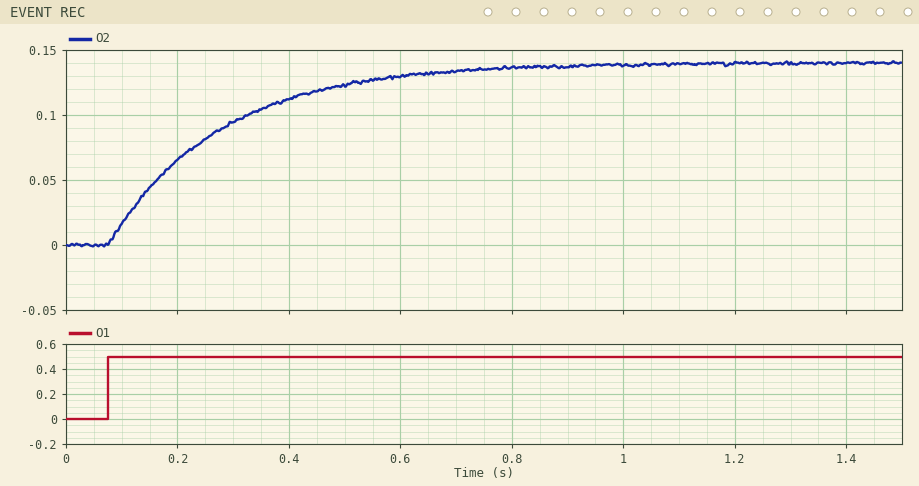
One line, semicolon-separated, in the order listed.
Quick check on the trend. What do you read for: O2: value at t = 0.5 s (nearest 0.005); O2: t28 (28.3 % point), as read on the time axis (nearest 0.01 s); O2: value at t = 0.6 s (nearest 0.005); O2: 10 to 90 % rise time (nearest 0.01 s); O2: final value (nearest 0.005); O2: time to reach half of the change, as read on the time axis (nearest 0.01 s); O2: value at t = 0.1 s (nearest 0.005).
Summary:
0.125; 0.14 s; 0.130; 0.44 s; 0.140; 0.21 s; 0.015
